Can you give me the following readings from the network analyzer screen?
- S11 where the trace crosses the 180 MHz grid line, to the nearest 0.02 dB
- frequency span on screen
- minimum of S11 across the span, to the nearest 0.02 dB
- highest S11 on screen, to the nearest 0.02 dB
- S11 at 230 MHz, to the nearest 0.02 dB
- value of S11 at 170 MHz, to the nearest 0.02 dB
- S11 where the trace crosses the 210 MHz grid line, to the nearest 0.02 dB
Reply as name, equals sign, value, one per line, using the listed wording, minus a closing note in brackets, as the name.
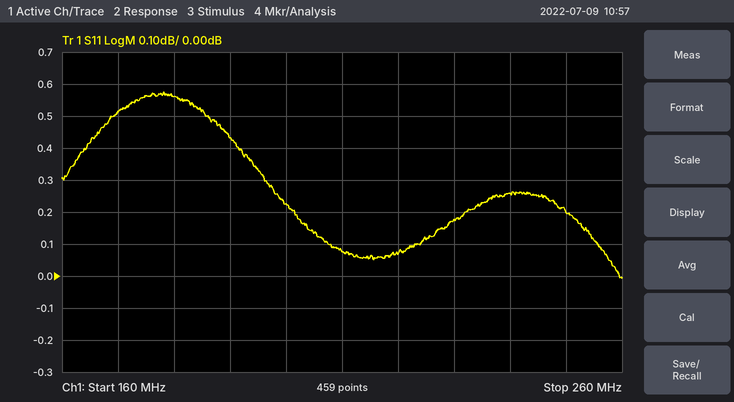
S11 where the trace crosses the 180 MHz grid line, to the nearest 0.02 dB = 0.56 dB
frequency span on screen = 100 MHz
minimum of S11 across the span, to the nearest 0.02 dB = 0.00 dB
highest S11 on screen, to the nearest 0.02 dB = 0.58 dB
S11 at 230 MHz, to the nearest 0.02 dB = 0.18 dB
value of S11 at 170 MHz, to the nearest 0.02 dB = 0.52 dB
S11 where the trace crosses the 210 MHz grid line, to the nearest 0.02 dB = 0.08 dB
